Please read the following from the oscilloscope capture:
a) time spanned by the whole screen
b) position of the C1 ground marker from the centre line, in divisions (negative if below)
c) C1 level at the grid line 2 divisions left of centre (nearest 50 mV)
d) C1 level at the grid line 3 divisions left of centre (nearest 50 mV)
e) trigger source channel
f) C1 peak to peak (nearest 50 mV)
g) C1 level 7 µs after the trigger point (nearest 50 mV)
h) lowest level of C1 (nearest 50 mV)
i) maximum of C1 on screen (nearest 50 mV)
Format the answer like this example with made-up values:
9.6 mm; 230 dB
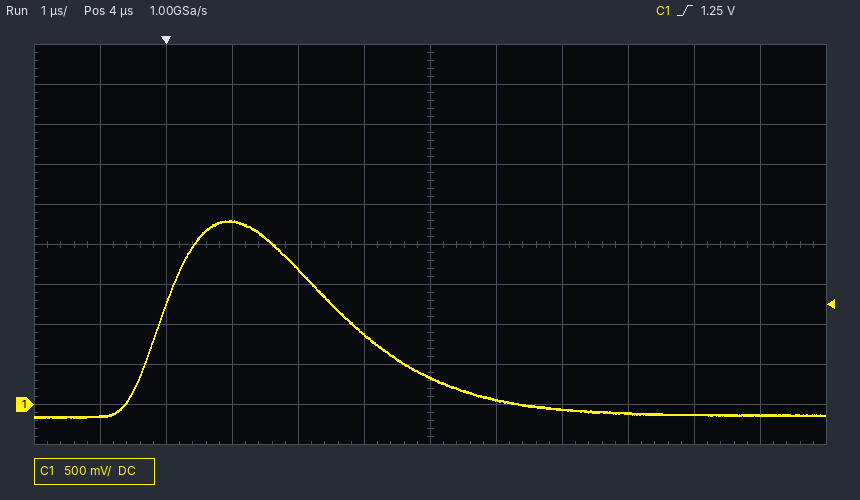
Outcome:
12 µs; -4.0 div; 1.70 V; 2.30 V; C1; 2.45 V; -100 mV; -150 mV; 2.30 V
